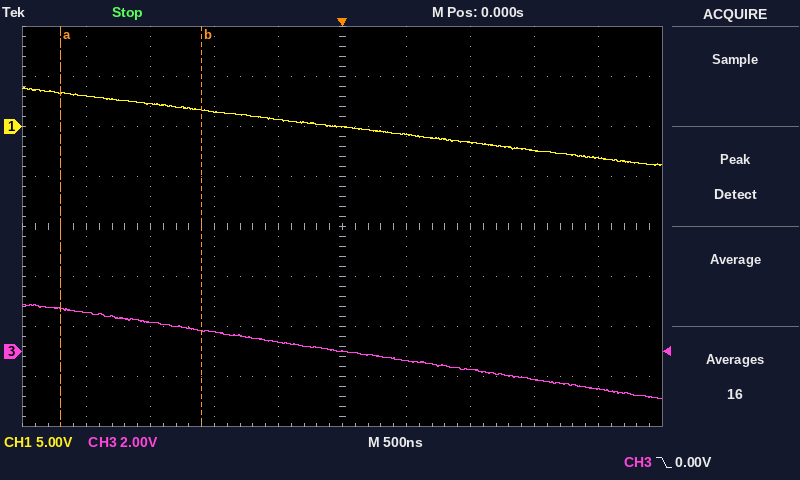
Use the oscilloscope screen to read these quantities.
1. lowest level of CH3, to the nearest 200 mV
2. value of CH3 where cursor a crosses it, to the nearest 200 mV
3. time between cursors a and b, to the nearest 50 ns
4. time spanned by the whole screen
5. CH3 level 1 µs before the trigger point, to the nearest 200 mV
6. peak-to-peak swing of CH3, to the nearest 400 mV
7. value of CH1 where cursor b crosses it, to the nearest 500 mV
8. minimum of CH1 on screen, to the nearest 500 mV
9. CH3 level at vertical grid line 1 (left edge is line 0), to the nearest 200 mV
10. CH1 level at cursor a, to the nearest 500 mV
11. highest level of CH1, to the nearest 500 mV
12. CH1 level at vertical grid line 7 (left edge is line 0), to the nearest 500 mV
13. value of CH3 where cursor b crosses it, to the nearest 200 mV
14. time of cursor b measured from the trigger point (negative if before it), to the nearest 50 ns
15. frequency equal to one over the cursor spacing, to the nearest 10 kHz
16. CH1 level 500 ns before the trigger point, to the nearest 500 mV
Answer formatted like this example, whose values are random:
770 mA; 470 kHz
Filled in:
-1.8 V; 1.8 V; 1.10 µs; 5 µs; 800 mV; 3.6 V; 1.5 V; -4.0 V; 1.6 V; 3.5 V; 4.0 V; -1.5 V; 800 mV; -1.10 µs; 910 kHz; 500 mV
